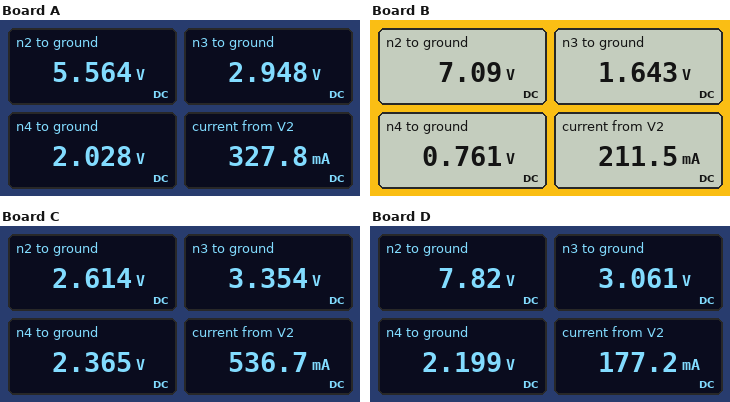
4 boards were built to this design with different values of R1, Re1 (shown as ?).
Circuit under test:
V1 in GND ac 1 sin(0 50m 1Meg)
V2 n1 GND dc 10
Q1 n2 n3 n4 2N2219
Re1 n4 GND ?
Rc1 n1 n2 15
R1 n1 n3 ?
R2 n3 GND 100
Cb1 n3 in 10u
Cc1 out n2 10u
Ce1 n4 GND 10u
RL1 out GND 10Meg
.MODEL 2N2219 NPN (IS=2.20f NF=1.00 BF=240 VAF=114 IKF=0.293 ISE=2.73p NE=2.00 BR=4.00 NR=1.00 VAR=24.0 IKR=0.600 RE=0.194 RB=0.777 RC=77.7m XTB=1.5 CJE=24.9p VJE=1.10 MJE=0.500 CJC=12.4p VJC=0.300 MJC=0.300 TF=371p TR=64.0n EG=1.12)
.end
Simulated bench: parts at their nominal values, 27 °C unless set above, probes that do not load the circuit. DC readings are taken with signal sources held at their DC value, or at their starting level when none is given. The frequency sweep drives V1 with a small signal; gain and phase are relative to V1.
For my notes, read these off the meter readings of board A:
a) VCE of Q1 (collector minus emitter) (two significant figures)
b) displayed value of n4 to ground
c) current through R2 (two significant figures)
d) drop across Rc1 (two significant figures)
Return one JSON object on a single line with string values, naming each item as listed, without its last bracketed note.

{"VCE of Q1 (collector minus emitter)": "3.5 V", "displayed value of n4 to ground": "2.028 V", "current through R2": "29 mA", "drop across Rc1": "4.4 V"}
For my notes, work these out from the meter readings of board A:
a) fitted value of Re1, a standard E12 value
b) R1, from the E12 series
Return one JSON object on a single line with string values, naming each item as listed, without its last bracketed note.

{"fitted value of Re1, a standard E12 value": "6.8 Ω", "R1, from the E12 series": "220 Ω"}
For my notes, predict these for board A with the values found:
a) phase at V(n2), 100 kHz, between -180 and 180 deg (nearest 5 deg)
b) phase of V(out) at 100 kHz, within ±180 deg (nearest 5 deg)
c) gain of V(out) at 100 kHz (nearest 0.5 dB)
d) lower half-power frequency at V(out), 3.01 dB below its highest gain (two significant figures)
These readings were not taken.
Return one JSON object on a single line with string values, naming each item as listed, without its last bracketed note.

{"phase at V(n2), 100 kHz, between -180 and 180 deg": "-155 deg", "phase of V(out) at 100 kHz, within ±180 deg": "-155 deg", "gain of V(out) at 100 kHz": "32.0 dB", "lower half-power frequency at V(out), 3.01 dB below its highest gain": "50 kHz"}
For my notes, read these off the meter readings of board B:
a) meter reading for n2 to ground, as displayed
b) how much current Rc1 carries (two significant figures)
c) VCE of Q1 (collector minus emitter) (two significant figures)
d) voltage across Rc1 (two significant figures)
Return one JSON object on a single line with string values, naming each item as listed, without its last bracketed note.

{"meter reading for n2 to ground, as displayed": "7.09 V", "how much current Rc1 carries": "190 mA", "VCE of Q1 (collector minus emitter)": "6.3 V", "voltage across Rc1": "2.9 V"}
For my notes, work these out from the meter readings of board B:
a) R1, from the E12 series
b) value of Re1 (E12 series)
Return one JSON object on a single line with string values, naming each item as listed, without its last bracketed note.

{"R1, from the E12 series": "470 Ω", "value of Re1": "3.9 Ω"}
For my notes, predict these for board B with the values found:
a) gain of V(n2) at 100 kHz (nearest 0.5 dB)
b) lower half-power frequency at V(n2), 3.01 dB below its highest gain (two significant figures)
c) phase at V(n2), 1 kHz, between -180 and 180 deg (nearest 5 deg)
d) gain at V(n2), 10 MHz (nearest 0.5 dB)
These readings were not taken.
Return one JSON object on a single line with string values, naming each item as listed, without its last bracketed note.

{"gain of V(n2) at 100 kHz": "31.0 dB", "lower half-power frequency at V(n2), 3.01 dB below its highest gain": "45 kHz", "phase at V(n2), 1 kHz, between -180 and 180 deg": "-155 deg", "gain at V(n2), 10 MHz": "31.5 dB"}
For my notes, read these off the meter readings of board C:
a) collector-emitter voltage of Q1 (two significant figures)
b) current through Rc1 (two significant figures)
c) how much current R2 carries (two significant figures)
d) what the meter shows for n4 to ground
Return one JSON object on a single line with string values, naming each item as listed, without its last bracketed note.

{"collector-emitter voltage of Q1": "250 mV", "current through Rc1": "490 mA", "how much current R2 carries": "34 mA", "what the meter shows for n4 to ground": "2.365 V"}
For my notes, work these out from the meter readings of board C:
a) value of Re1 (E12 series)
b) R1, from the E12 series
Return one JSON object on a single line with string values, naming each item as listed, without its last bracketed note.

{"value of Re1": "4.7 Ω", "R1, from the E12 series": "150 Ω"}
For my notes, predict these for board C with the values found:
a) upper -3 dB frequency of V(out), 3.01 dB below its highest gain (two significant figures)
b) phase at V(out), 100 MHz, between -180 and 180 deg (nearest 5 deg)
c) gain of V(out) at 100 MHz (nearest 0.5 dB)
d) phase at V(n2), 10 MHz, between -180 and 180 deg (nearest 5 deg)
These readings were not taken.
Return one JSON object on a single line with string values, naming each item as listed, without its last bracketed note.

{"upper -3 dB frequency of V(out), 3.01 dB below its highest gain": "850 kHz", "phase at V(out), 100 MHz, between -180 and 180 deg": "5 deg", "gain of V(out) at 100 MHz": "-11.5 dB", "phase at V(n2), 10 MHz, between -180 and 180 deg": "55 deg"}
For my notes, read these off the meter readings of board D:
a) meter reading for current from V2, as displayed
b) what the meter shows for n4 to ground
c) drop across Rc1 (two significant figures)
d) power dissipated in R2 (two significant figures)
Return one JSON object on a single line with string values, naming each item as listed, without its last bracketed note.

{"meter reading for current from V2, as displayed": "177.2 mA", "what the meter shows for n4 to ground": "2.199 V", "drop across Rc1": "2.2 V", "power dissipated in R2": "94 mW"}
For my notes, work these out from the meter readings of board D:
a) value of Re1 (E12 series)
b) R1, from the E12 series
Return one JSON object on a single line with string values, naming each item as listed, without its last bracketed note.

{"value of Re1": "15 Ω", "R1, from the E12 series": "220 Ω"}
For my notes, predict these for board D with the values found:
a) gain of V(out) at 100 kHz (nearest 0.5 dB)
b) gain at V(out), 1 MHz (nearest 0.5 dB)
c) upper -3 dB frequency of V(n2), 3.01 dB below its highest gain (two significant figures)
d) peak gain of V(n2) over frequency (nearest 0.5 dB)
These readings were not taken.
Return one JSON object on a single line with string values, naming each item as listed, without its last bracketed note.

{"gain of V(out) at 100 kHz": "30.0 dB", "gain at V(out), 1 MHz": "30.5 dB", "upper -3 dB frequency of V(n2), 3.01 dB below its highest gain": "160 MHz", "peak gain of V(n2) over frequency": "30.5 dB"}
